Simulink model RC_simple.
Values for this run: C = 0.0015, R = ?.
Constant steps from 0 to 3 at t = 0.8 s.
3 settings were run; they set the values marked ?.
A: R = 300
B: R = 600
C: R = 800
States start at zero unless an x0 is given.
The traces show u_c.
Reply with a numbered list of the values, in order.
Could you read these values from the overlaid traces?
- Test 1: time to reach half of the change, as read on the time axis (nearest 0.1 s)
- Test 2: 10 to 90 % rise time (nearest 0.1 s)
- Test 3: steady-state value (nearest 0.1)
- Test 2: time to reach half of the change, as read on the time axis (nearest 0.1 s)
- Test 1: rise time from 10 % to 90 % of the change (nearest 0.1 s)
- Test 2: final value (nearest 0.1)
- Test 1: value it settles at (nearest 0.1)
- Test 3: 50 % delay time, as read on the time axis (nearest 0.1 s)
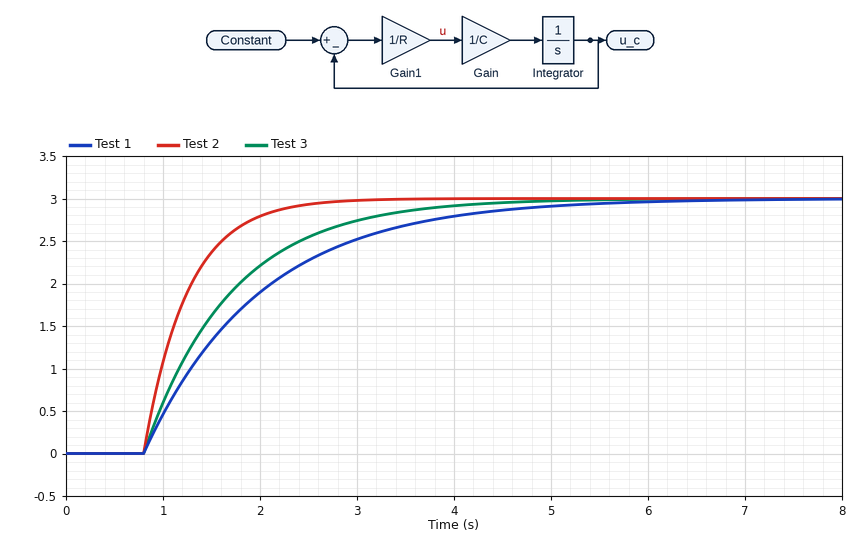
1. 1.6 s
2. 1.0 s
3. 3.0
4. 1.1 s
5. 2.6 s
6. 3.0
7. 3.0
8. 1.4 s
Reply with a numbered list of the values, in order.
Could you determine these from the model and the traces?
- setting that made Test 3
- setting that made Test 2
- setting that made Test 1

1. B
2. A
3. C
